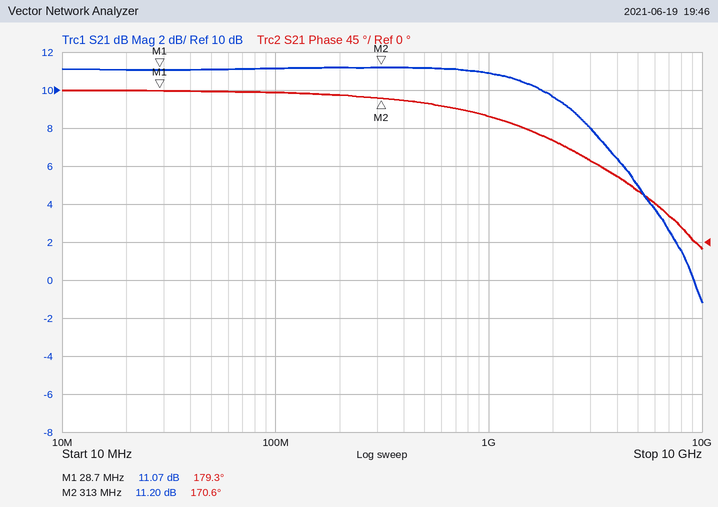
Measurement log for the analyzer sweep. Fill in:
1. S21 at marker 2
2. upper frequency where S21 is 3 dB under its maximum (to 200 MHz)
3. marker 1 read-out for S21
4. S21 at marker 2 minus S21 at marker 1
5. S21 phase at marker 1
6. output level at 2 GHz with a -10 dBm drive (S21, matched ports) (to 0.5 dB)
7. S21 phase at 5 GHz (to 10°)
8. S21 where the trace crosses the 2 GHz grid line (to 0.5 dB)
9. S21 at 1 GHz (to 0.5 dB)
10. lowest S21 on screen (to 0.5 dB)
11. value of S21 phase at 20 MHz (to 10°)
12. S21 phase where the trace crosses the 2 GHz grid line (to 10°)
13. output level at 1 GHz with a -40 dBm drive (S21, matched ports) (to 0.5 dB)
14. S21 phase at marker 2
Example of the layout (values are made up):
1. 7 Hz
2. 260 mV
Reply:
1. 11.20 dB
2. 2.8 GHz
3. 11.07 dB
4. 0.13 dB
5. 179.3°
6. -0.5 dBm
7. 60°
8. 9.5 dB
9. 11.0 dB
10. -1.0 dB
11. 180°
12. 120°
13. -29.0 dBm
14. 170.6°
